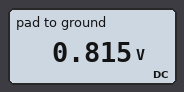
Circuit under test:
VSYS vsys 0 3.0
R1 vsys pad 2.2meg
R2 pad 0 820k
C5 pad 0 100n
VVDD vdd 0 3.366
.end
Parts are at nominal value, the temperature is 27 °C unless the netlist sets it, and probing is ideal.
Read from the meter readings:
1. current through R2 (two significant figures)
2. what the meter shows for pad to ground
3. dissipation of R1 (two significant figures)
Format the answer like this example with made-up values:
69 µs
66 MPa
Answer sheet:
990 nA
0.815 V
2.2 µW
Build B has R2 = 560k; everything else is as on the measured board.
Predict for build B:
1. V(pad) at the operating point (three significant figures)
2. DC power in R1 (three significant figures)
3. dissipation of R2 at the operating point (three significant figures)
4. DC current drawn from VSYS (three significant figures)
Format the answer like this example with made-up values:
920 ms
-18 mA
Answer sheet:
609 mV
2.60 µW
662 nW
1.09 µA
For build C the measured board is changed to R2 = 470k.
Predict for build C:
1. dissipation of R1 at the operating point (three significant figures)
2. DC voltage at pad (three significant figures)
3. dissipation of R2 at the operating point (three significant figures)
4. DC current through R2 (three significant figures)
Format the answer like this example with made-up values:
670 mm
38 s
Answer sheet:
2.78 µW
528 mV
593 nW
1.12 µA
